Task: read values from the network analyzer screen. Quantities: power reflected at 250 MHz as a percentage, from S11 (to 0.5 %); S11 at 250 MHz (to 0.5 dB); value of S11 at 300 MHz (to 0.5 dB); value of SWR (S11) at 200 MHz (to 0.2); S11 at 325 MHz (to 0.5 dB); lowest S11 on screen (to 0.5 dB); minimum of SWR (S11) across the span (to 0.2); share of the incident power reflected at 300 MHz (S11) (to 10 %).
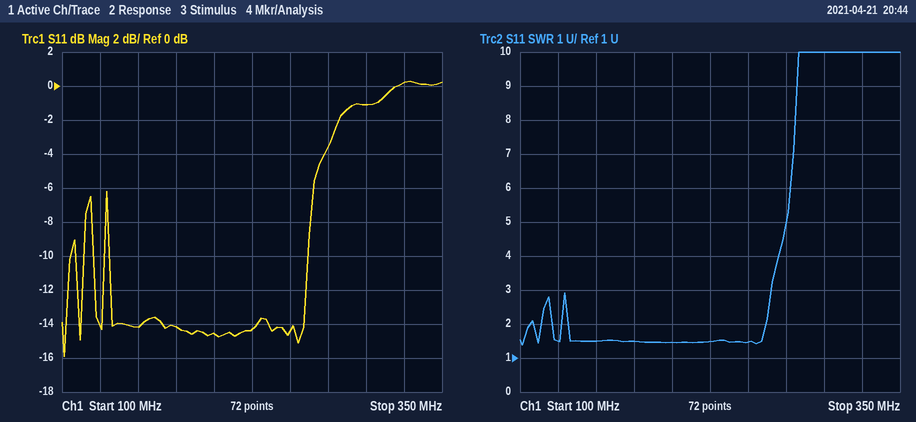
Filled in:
3.5 %
-14.5 dB
-1.0 dB
1.4
0.0 dB
-16.0 dB
1.4
80 %
